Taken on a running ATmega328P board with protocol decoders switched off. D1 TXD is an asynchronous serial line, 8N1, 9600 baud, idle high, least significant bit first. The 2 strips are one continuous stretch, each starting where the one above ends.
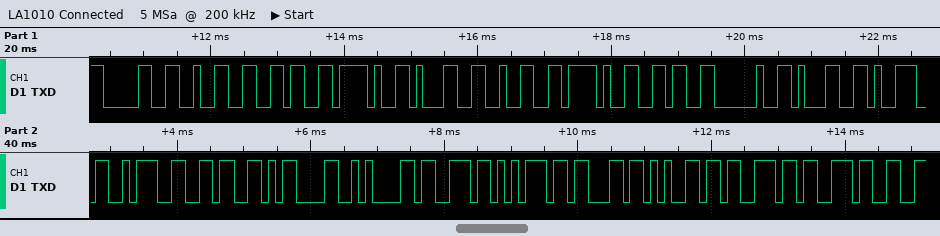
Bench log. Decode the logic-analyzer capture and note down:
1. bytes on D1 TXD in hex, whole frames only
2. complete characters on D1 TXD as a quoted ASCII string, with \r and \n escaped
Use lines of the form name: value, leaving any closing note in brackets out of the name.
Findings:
bytes on D1 TXD in hex, whole frames only: 30 32 36 2F 31 32 2F 36 20 31 39 3A 36 0D 0A 73 75 63 65 73 73
complete characters on D1 TXD as a quoted ASCII string, with \r and \n escaped: "026/12/6 19:6\r\nsucess"
